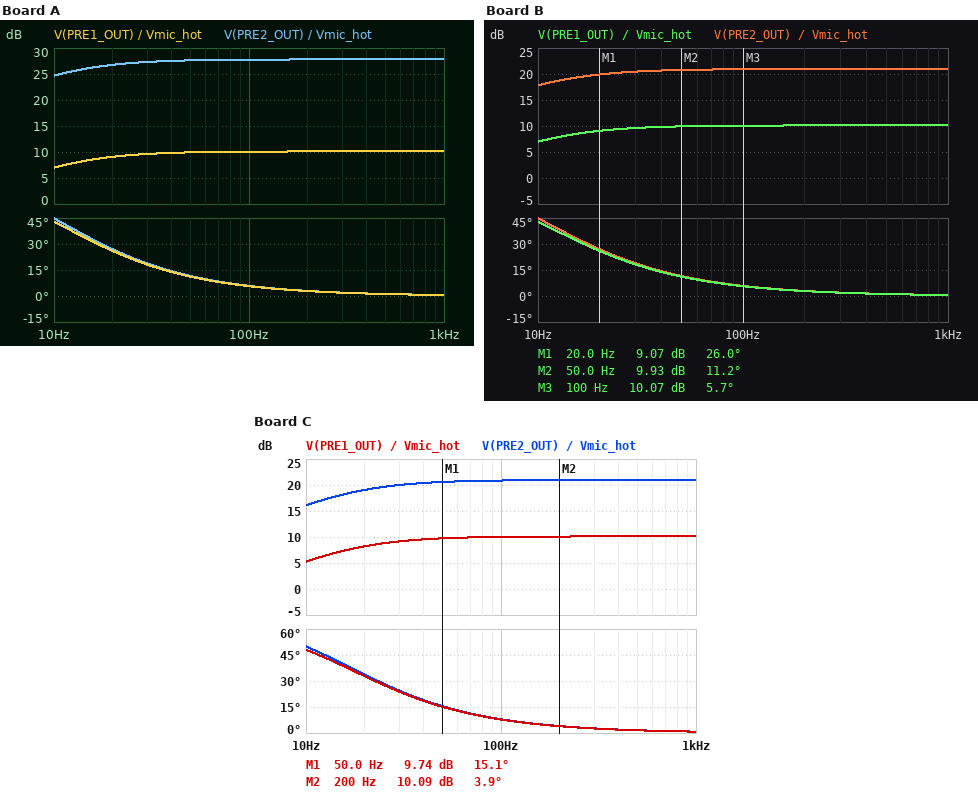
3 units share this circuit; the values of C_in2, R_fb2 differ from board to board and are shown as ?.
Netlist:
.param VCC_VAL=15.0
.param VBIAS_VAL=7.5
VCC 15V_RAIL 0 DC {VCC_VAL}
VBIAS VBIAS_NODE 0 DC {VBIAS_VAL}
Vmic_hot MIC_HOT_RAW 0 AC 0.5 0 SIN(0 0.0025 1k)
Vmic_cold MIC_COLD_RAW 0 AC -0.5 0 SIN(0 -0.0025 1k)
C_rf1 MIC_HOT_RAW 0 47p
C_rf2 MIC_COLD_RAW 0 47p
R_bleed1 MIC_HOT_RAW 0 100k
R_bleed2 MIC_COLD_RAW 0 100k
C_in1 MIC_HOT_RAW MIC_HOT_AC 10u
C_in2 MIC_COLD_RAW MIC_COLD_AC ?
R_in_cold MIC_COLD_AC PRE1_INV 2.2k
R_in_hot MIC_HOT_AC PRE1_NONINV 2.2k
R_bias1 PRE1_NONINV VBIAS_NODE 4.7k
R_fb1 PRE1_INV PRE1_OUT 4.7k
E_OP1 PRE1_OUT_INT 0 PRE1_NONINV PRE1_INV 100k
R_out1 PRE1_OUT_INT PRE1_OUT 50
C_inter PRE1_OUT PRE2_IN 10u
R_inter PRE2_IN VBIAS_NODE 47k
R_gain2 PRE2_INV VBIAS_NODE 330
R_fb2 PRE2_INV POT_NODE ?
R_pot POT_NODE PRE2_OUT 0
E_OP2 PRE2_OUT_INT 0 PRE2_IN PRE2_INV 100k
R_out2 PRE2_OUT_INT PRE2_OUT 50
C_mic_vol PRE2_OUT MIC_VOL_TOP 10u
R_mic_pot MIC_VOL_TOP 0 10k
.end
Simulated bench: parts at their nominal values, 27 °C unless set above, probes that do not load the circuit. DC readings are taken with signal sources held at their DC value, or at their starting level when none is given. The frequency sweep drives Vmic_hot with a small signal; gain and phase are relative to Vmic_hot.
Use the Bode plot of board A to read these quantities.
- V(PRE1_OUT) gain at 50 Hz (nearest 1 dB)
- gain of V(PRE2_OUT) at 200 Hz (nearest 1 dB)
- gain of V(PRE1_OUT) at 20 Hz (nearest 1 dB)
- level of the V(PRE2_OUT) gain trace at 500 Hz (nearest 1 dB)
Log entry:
10 dB
28 dB
9 dB
28 dB
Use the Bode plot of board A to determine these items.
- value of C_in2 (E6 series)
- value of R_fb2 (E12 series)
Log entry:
6.8 µF
2.2 kΩ
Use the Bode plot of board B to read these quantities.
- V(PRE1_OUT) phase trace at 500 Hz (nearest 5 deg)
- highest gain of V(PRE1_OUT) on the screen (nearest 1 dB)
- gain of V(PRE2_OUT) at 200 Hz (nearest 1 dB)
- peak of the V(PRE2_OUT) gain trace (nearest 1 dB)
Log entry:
0 deg
10 dB
21 dB
21 dB
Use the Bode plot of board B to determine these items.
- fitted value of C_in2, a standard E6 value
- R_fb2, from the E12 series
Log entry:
6.8 µF
820 Ω
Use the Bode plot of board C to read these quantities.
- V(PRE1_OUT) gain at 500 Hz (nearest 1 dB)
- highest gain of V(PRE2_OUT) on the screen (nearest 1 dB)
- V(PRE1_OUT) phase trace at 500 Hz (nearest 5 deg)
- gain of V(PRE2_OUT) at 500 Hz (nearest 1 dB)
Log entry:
10 dB
21 dB
0 deg
21 dB
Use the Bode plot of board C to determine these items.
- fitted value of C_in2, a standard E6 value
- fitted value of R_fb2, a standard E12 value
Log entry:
4.7 µF
820 Ω
